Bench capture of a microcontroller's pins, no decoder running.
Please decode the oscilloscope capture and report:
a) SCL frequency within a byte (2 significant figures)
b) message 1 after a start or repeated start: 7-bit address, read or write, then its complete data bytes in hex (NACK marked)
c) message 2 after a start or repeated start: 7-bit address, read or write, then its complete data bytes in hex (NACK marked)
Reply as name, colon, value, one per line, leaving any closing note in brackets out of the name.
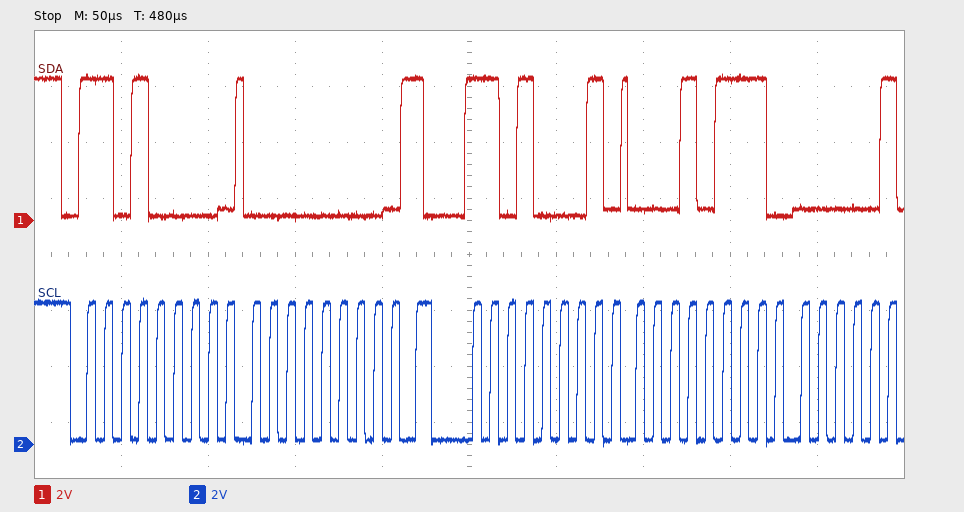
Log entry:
SCL frequency within a byte: 100 kHz
message 1 after a start or repeated start: 7-bit address, read or write, then its complete data bytes in hex: 0x68 write: 00
message 2 after a start or repeated start: 7-bit address, read or write, then its complete data bytes in hex: 0x68 read: 17
